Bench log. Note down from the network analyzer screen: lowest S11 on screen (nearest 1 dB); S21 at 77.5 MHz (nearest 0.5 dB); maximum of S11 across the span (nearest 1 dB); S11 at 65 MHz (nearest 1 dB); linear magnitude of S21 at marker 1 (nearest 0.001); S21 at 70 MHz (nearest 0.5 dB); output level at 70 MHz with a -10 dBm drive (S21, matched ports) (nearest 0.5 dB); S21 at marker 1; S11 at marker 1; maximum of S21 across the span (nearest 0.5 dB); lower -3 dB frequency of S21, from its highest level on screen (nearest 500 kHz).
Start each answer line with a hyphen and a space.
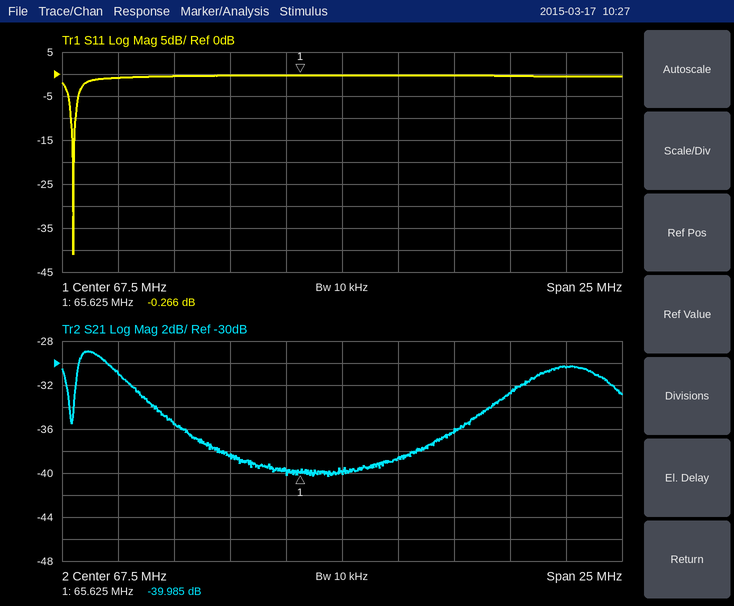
- -41 dB
- -30.5 dB
- 0 dB
- 0 dB
- 0.010
- -38.5 dB
- -48.5 dBm
- -39.985 dB
- -0.266 dB
- -29.0 dB
- 55.5 MHz
